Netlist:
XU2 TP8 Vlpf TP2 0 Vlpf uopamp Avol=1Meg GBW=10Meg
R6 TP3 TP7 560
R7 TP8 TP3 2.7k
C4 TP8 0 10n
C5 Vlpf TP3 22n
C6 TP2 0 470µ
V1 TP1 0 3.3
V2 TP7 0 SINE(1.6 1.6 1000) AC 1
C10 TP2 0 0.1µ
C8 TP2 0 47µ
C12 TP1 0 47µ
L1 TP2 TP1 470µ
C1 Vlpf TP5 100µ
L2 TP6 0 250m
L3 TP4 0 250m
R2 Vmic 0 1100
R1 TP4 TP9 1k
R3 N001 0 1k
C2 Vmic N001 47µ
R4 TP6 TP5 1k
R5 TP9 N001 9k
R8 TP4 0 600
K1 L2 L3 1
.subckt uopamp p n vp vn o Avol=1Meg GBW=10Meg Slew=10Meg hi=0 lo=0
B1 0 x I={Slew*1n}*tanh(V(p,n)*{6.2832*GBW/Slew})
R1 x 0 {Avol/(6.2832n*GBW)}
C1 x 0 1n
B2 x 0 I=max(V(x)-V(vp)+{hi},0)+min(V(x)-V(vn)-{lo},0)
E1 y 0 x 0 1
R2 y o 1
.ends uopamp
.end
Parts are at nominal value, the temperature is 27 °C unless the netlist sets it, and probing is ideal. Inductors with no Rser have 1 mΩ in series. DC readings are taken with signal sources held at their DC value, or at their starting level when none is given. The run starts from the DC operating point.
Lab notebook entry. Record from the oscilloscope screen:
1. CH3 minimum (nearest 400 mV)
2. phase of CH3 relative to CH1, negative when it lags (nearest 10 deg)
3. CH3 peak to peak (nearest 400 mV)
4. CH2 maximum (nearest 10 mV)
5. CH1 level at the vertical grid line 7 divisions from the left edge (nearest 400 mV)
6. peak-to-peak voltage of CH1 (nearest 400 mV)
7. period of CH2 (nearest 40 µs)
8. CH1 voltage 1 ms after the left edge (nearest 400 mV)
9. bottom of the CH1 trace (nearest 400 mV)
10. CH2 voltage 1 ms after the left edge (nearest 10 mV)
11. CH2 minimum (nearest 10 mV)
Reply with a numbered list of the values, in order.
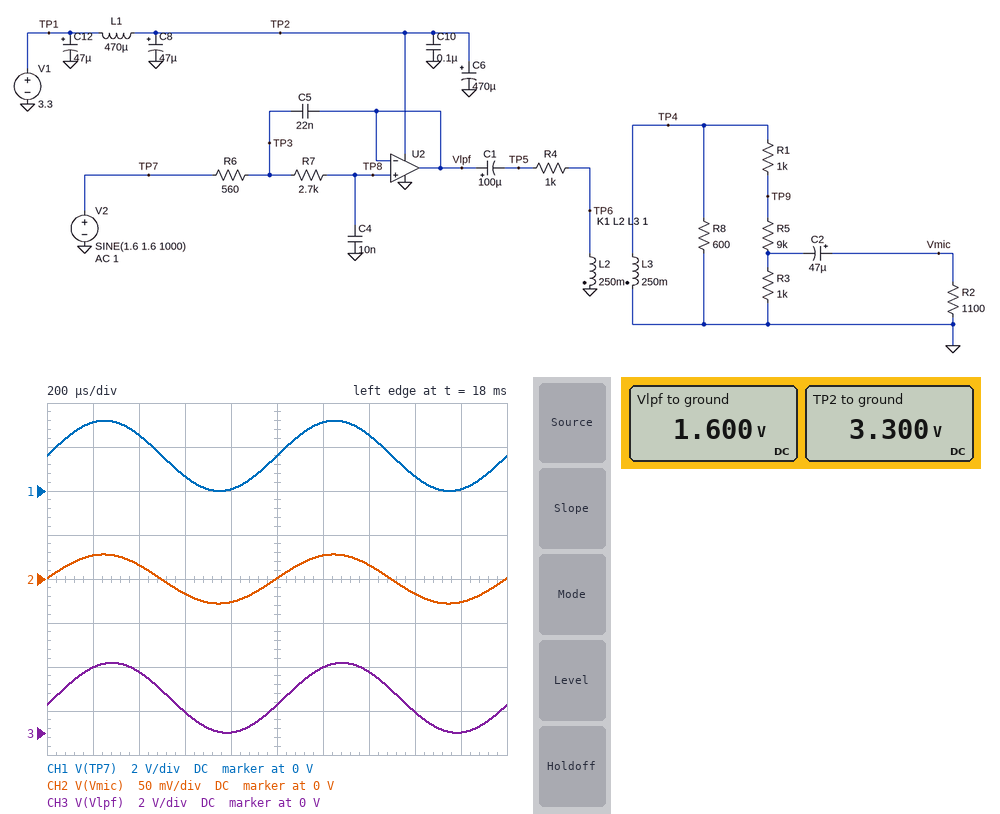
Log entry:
1. 0 V
2. -10 deg
3. 3.2 V
4. 30 mV
5. 2.4 V
6. 3.2 V
7. 1.00 ms
8. 1.6 V
9. 0 V
10. 0 V
11. -30 mV
